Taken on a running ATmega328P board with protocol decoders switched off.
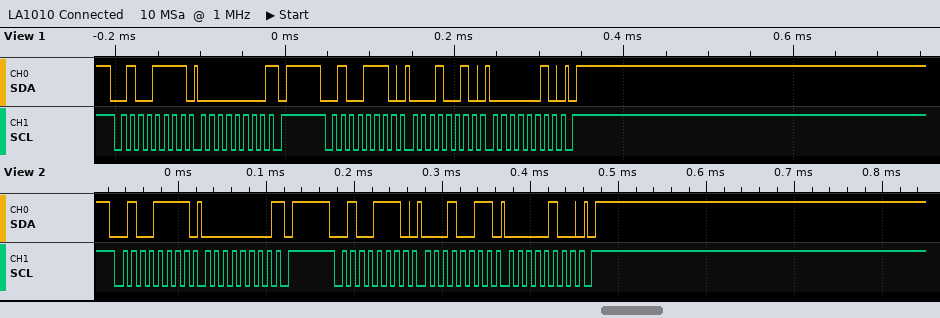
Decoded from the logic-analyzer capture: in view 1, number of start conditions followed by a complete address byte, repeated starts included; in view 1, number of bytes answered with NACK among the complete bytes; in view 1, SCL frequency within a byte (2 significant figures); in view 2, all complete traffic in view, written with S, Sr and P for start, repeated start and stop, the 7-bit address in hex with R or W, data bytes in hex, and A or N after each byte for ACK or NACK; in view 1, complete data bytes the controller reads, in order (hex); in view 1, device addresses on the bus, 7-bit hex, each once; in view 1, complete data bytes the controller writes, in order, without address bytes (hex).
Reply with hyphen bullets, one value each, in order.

- 2
- 1
- 100 kHz
- S 27R A 00 N P S 27W A 13 A 04 A P
- 00
- 0x27
- 12 02
